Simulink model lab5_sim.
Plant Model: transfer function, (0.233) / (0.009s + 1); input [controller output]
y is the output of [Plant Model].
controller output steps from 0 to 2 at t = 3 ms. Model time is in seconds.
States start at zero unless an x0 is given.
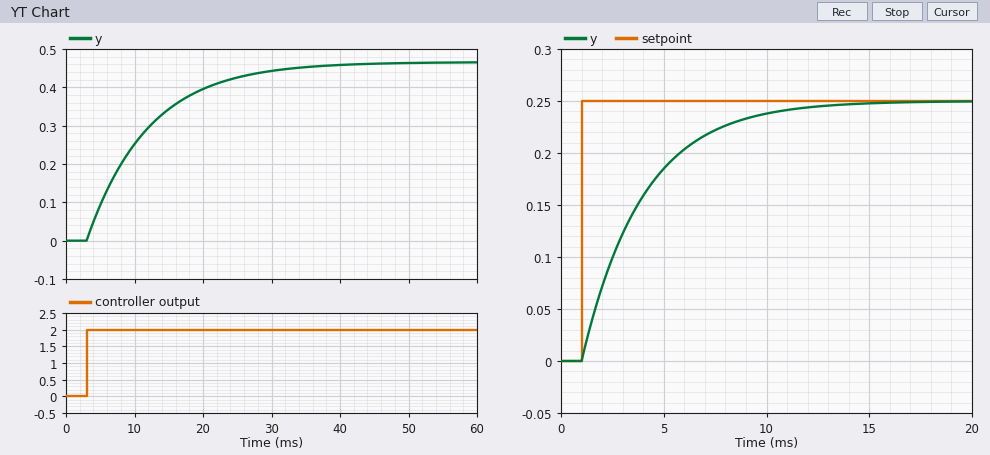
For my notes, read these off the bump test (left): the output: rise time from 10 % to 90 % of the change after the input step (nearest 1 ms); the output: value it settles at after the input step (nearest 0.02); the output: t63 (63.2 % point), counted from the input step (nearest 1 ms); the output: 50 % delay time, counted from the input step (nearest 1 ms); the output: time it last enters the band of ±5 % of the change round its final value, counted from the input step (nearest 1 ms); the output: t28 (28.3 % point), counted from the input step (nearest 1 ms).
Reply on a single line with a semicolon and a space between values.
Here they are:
20 ms; 0.46; 9 ms; 6 ms; 27 ms; 3 ms
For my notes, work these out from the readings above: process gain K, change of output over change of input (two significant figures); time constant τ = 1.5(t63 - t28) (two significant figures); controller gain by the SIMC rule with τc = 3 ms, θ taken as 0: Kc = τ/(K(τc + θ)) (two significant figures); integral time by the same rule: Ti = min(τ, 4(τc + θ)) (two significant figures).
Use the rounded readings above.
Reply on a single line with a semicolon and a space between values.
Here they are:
0.23; 9.0 ms; 13; 9.0 ms
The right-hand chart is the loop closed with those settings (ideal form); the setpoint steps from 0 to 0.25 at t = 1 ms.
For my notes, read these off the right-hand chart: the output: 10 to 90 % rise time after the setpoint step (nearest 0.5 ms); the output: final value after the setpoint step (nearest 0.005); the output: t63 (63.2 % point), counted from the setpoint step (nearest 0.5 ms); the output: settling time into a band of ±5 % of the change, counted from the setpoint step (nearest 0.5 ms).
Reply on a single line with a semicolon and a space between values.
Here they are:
6.5 ms; 0.250; 3.0 ms; 9.0 ms
